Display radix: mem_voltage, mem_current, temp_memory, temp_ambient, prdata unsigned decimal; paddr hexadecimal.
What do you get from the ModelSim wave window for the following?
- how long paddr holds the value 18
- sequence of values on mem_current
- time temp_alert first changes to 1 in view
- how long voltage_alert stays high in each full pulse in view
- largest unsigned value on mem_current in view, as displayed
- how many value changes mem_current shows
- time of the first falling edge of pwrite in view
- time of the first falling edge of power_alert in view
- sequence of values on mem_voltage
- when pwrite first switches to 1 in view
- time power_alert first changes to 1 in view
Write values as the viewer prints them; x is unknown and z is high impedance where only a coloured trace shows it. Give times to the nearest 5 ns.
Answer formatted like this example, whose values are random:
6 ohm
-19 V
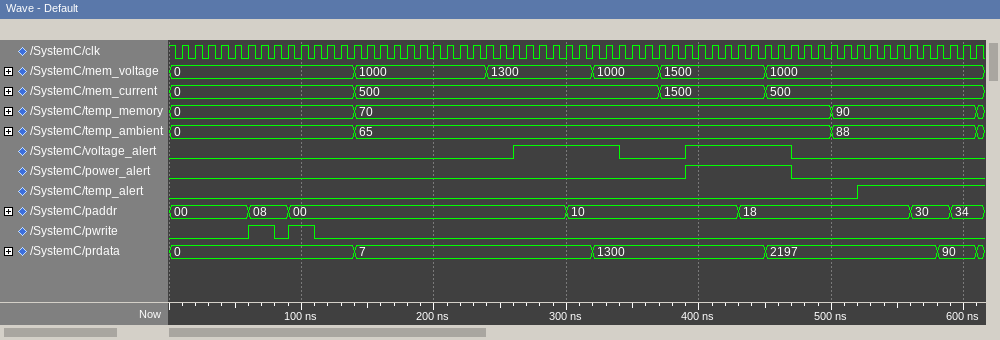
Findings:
130 ns
0, 500, 1500, 500
520 ns
80 ns, 80 ns
1500
3
80 ns
470 ns
0, 1000, 1300, 1000, 1500, 1000
60 ns
390 ns
